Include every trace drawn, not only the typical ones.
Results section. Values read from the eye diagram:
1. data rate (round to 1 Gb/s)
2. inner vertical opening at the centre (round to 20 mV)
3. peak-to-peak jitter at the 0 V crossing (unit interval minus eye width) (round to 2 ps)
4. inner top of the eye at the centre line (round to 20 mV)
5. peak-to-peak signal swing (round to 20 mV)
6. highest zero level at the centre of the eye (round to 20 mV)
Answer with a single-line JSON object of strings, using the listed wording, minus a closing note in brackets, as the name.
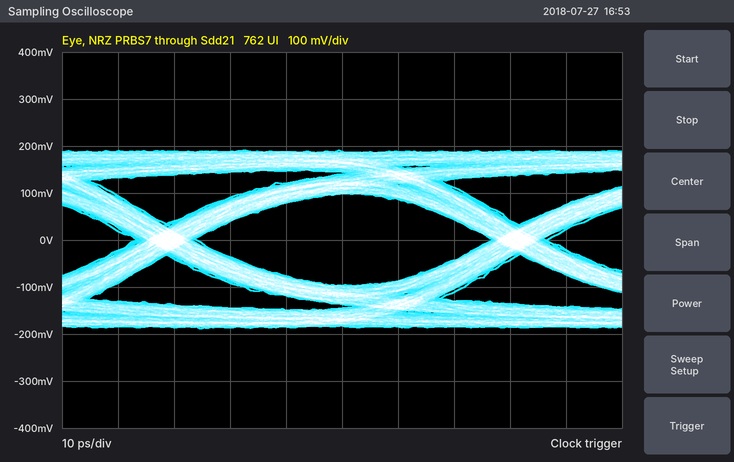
{"data rate": "16 Gb/s", "inner vertical opening at the centre": "200 mV", "peak-to-peak jitter at the 0 V crossing (unit interval minus eye width)": "10 ps", "inner top of the eye at the centre line": "100 mV", "peak-to-peak signal swing": "380 mV", "highest zero level at the centre of the eye": "-100 mV"}
